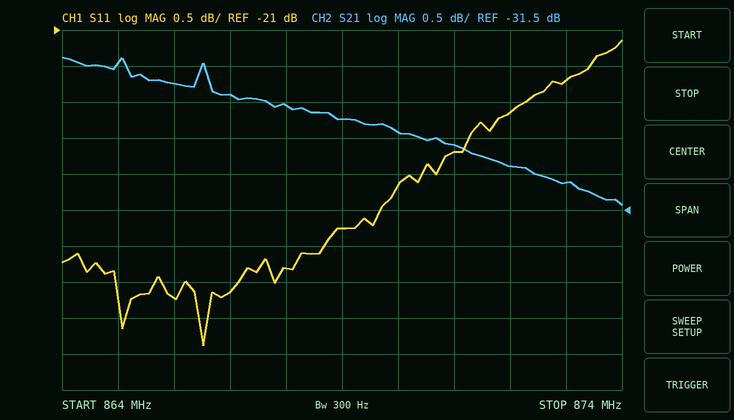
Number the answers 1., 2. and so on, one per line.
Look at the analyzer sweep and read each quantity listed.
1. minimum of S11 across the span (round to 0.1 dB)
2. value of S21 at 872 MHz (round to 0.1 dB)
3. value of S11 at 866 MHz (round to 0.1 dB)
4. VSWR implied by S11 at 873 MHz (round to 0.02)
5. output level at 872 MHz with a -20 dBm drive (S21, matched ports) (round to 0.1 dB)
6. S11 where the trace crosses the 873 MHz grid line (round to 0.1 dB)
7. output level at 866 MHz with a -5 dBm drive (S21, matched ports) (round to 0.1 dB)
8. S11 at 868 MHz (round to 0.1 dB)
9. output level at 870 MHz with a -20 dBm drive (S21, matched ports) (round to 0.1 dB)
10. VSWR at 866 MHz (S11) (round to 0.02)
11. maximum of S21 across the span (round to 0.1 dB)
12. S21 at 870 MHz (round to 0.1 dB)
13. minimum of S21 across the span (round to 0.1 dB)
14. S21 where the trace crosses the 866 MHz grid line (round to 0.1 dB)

1. -25.4 dB
2. -30.9 dB
3. -24.7 dB
4. 1.18
5. -50.9 dBm
6. -21.7 dB
7. -34.7 dBm
8. -24.3 dB
9. -50.4 dBm
10. 1.12
11. -29.4 dB
12. -30.4 dB
13. -31.4 dB
14. -29.7 dB
